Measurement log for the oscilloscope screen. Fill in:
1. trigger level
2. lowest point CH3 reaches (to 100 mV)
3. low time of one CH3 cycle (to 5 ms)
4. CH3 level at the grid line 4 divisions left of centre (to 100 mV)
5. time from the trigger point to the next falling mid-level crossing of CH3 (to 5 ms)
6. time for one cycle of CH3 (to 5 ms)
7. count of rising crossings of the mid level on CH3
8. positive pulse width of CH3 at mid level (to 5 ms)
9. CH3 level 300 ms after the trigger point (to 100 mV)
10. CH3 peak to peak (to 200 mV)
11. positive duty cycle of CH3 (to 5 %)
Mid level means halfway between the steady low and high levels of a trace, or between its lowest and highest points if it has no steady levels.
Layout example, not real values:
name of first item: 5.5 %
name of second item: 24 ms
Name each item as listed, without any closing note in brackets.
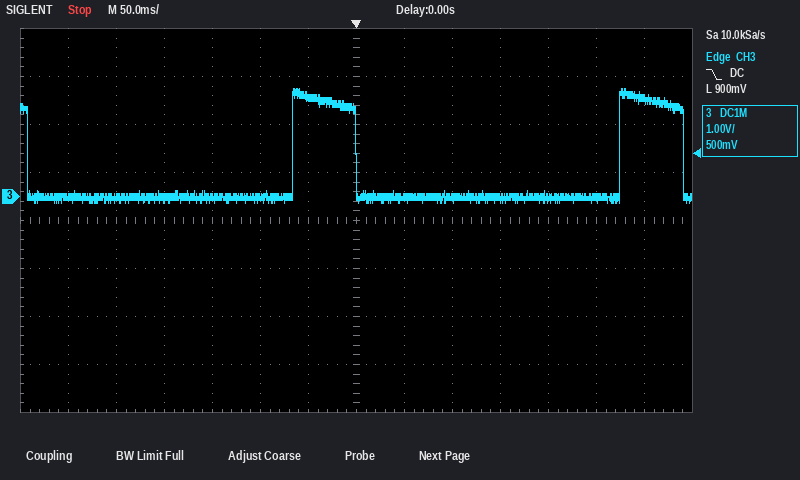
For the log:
trigger level: 900 mV
lowest point CH3 reaches: -100 mV
low time of one CH3 cycle: 275 ms
CH3 level at the grid line 4 divisions left of centre: 0.0 V
time from the trigger point to the next falling mid-level crossing of CH3: 340 ms
time for one cycle of CH3: 340 ms
count of rising crossings of the mid level on CH3: 2
positive pulse width of CH3 at mid level: 65 ms
CH3 level 300 ms after the trigger point: 2.0 V
CH3 peak to peak: 2.4 V
positive duty cycle of CH3: 20 %
